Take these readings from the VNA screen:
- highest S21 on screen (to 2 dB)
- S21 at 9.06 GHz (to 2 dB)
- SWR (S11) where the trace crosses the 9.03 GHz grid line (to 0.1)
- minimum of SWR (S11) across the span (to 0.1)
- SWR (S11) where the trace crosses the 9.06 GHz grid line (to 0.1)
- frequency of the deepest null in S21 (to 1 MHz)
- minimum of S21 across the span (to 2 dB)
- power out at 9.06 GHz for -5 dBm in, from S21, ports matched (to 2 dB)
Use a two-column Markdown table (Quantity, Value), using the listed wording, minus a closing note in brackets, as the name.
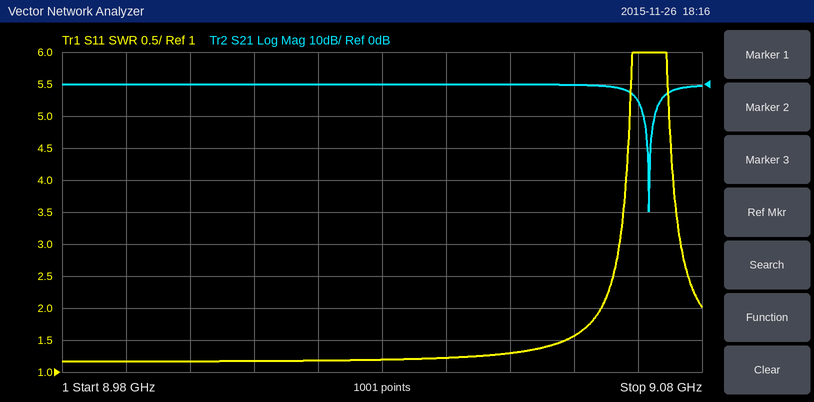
| Quantity | Value |
|---|---|
| highest S21 on screen | 0 dB |
| S21 at 9.06 GHz | 0 dB |
| SWR (S11) where the trace crosses the 9.03 GHz grid line | 1.2 |
| minimum of SWR (S11) across the span | 1.2 |
| SWR (S11) where the trace crosses the 9.06 GHz grid line | 1.6 |
| frequency of the deepest null in S21 | 9.072 GHz |
| minimum of S21 across the span | -40 dB |
| power out at 9.06 GHz for -5 dBm in, from S21, ports matched | -6 dBm |
